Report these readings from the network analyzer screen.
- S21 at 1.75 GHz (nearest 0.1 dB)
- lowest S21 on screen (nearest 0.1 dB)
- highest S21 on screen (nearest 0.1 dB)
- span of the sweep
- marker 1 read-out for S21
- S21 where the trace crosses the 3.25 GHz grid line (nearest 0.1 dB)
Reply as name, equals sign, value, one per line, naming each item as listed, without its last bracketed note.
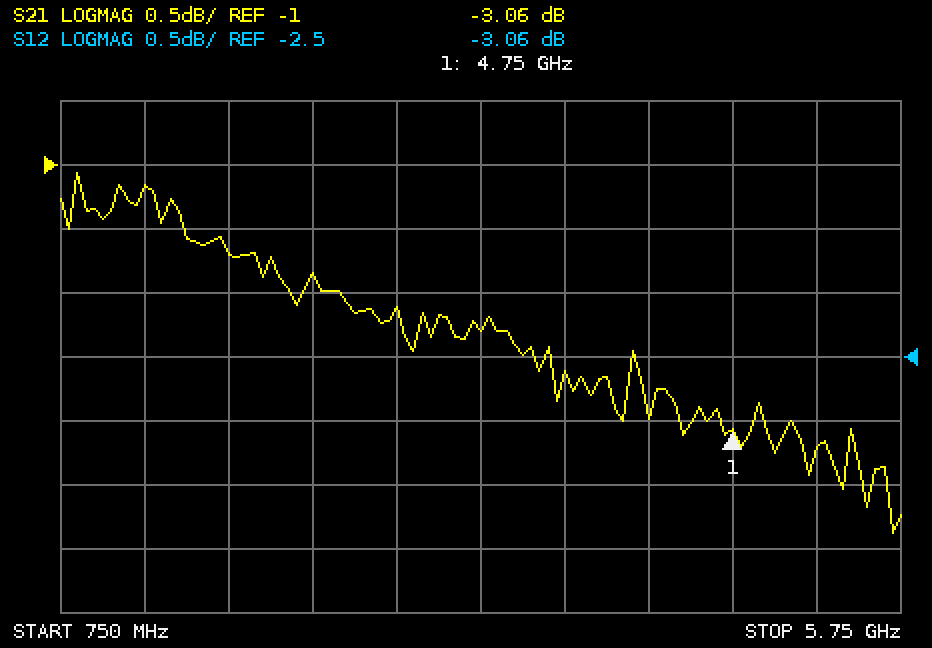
S21 at 1.75 GHz = -1.7 dB
lowest S21 on screen = -3.9 dB
highest S21 on screen = -1.1 dB
span of the sweep = 5 GHz
marker 1 read-out for S21 = -3.06 dB
S21 where the trace crosses the 3.25 GHz grid line = -2.3 dB
